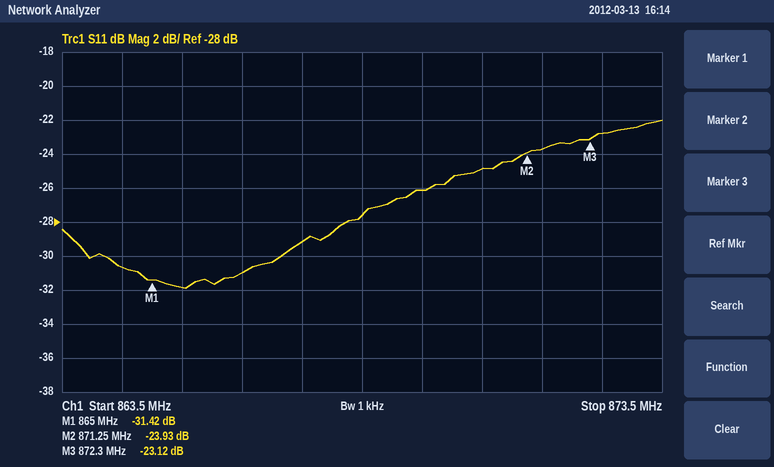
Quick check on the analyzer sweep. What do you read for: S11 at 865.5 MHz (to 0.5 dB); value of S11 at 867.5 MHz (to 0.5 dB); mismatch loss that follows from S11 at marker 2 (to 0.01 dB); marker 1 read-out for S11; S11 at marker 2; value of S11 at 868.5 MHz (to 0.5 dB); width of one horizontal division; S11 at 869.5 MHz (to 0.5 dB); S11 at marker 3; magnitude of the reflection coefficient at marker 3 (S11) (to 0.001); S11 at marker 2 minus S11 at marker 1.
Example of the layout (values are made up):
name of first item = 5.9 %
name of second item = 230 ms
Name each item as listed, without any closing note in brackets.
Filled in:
S11 at 865.5 MHz = -32.0 dB
value of S11 at 867.5 MHz = -29.0 dB
mismatch loss that follows from S11 at marker 2 = 0.02 dB
marker 1 read-out for S11 = -31.42 dB
S11 at marker 2 = -23.93 dB
value of S11 at 868.5 MHz = -27.5 dB
width of one horizontal division = 1 MHz
S11 at 869.5 MHz = -26.0 dB
S11 at marker 3 = -23.12 dB
magnitude of the reflection coefficient at marker 3 (S11) = 0.070
S11 at marker 2 minus S11 at marker 1 = 7.49 dB
